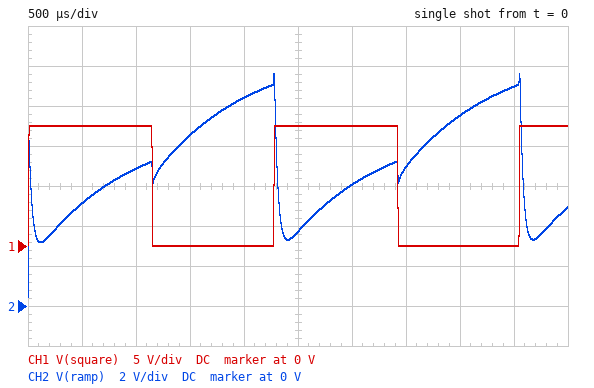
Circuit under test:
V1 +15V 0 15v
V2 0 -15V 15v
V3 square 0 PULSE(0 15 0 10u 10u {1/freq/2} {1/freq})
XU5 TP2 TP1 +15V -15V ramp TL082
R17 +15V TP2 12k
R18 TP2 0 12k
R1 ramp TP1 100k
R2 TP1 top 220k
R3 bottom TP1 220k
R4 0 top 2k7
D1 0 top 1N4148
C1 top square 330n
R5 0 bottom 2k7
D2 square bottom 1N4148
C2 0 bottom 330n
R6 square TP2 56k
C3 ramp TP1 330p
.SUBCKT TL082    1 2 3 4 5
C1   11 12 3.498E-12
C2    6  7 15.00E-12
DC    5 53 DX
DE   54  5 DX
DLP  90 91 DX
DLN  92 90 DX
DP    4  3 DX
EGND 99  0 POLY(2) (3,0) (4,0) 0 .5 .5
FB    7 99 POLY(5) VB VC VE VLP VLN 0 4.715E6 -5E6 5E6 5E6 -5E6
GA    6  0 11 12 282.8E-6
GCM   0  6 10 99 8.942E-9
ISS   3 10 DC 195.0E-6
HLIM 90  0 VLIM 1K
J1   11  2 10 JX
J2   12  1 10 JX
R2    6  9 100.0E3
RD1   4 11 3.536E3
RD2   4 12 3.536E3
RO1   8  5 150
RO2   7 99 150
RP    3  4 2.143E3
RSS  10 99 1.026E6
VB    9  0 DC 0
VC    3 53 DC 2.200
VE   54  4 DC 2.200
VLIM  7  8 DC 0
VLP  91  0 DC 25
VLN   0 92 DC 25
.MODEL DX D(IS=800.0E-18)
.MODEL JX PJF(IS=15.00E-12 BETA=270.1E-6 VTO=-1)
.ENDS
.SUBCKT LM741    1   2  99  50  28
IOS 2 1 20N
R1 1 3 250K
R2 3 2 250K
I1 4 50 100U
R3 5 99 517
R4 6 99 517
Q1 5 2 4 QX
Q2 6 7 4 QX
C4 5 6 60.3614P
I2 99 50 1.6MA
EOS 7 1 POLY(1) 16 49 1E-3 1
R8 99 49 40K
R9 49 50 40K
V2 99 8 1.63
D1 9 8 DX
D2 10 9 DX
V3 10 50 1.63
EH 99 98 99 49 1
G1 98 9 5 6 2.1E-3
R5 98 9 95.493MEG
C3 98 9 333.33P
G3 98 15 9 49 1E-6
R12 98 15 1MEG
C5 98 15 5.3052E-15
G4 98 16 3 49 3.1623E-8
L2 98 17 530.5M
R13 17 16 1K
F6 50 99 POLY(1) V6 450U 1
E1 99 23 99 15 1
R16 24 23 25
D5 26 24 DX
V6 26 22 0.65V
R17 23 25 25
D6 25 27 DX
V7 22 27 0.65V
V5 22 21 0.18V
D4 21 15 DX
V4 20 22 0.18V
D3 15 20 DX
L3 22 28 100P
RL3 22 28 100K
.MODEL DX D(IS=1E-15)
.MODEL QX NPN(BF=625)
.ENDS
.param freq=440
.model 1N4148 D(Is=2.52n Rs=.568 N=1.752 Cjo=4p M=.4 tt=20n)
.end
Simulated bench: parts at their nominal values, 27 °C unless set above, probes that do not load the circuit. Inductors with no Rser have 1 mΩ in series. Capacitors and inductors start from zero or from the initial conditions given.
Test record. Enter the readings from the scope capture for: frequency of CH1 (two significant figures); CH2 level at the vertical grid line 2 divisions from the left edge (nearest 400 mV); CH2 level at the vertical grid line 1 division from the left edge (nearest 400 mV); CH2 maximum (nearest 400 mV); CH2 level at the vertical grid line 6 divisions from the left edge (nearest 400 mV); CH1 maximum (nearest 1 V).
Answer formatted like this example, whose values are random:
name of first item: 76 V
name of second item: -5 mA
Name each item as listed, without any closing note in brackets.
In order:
frequency of CH1: 440 Hz
CH2 level at the vertical grid line 2 divisions from the left edge: 6.8 V
CH2 level at the vertical grid line 1 division from the left edge: 5.2 V
CH2 maximum: 11.6 V
CH2 level at the vertical grid line 6 divisions from the left edge: 6.0 V
CH1 maximum: 15 V
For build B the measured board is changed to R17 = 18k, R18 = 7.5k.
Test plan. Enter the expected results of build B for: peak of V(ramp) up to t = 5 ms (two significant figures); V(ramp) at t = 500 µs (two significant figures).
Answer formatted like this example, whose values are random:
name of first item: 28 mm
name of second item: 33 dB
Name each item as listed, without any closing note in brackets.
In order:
peak of V(ramp) up to t = 5 ms: 6.3 V
V(ramp) at t = 500 µs: -400 mV
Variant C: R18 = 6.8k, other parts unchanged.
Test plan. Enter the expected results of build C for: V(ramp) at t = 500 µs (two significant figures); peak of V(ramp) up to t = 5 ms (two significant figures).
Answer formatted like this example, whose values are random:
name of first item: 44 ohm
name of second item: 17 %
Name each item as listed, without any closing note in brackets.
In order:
V(ramp) at t = 500 µs: 1.1 V
peak of V(ramp) up to t = 5 ms: 8.1 V
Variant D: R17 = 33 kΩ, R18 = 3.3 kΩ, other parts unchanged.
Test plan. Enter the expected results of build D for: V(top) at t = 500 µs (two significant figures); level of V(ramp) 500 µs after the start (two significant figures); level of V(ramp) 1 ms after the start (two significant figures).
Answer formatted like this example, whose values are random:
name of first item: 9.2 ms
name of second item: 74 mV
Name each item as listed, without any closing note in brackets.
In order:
V(top) at t = 500 µs: 8.6 V
level of V(ramp) 500 µs after the start: -6.6 V
level of V(ramp) 1 ms after the start: -4.9 V
